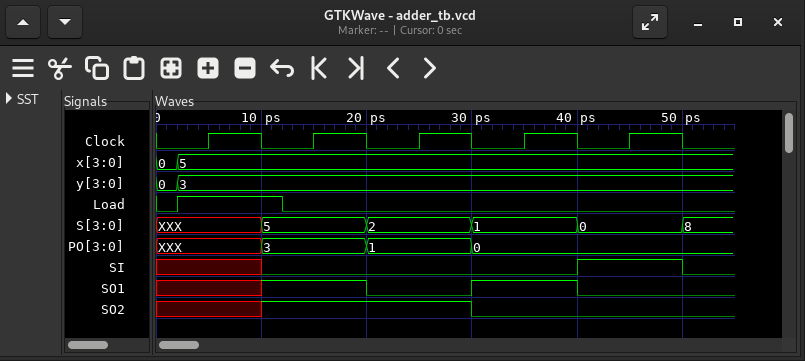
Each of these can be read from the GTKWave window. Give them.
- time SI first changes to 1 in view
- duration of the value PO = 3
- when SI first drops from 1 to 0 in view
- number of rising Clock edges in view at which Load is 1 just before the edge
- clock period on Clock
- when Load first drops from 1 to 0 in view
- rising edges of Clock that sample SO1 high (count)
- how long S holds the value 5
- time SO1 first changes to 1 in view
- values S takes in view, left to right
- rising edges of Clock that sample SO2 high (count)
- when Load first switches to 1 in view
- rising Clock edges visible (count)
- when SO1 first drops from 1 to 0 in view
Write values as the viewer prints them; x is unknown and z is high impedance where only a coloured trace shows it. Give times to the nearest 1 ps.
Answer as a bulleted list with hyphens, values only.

- 40 ps
- 10 ps
- 50 ps
- 1
- 10 ps
- 12 ps
- 2
- 10 ps
- 10 ps
- XXX, 5, 2, 1, 0, 8
- 2
- 2 ps
- 5
- 20 ps
